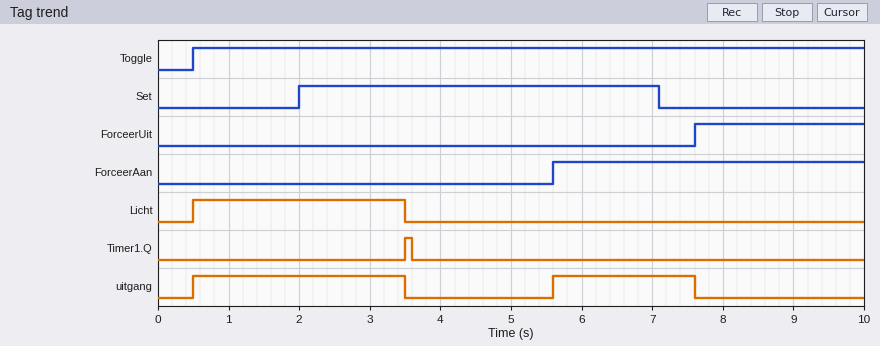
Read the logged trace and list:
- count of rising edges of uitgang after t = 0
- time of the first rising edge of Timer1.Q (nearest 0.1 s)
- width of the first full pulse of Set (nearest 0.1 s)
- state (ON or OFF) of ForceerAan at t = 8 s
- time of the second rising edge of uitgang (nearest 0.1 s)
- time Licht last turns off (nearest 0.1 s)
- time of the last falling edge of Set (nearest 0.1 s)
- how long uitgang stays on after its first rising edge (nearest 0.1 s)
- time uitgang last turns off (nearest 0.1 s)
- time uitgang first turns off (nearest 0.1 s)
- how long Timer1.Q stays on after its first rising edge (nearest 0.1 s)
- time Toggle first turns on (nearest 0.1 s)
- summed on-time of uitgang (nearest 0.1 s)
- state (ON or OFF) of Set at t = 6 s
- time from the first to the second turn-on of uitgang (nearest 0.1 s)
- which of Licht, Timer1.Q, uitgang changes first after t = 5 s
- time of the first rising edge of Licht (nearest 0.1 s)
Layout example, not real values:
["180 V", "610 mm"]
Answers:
["2", "3.5 s", "5.1 s", "ON", "5.6 s", "3.5 s", "7.1 s", "3.0 s", "7.6 s", "3.5 s", "0.1 s", "0.5 s", "5.0 s", "ON", "5.1 s", "uitgang", "0.5 s"]
